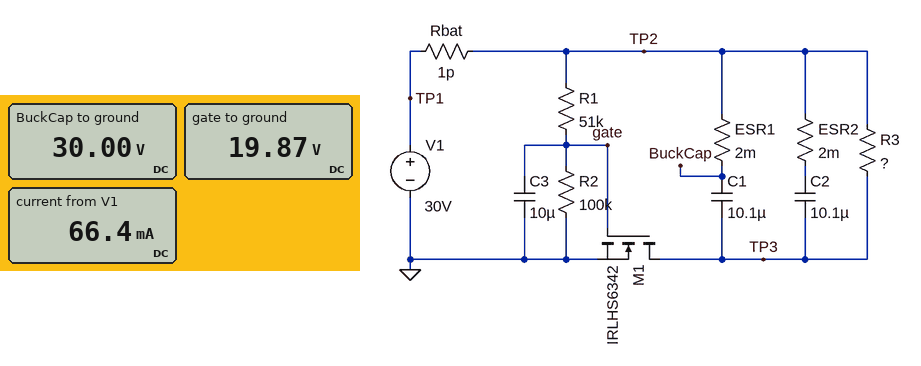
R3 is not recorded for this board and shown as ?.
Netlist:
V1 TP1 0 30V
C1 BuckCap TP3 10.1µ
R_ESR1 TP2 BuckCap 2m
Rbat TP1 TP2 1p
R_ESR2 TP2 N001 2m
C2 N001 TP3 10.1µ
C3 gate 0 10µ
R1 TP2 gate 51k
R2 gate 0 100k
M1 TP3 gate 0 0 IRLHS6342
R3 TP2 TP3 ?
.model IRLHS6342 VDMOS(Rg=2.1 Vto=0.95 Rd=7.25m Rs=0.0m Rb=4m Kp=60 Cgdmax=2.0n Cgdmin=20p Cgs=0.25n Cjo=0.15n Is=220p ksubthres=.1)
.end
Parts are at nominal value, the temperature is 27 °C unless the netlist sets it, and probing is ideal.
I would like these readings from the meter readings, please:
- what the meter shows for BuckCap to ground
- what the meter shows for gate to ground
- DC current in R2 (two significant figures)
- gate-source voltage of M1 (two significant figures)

30.00 V
19.87 V
200 µA
20 V
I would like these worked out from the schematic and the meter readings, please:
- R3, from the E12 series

470 Ω
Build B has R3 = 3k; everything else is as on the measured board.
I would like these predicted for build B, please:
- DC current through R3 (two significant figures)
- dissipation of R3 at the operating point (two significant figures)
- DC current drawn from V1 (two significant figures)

10 mA
300 mW
16 mA
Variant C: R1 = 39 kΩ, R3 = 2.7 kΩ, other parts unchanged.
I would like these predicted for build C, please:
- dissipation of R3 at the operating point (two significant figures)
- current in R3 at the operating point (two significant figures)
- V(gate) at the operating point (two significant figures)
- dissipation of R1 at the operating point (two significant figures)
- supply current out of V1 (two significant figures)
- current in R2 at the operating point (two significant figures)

330 mW
11 mA
22 V
1.8 mW
16 mA
220 µA
